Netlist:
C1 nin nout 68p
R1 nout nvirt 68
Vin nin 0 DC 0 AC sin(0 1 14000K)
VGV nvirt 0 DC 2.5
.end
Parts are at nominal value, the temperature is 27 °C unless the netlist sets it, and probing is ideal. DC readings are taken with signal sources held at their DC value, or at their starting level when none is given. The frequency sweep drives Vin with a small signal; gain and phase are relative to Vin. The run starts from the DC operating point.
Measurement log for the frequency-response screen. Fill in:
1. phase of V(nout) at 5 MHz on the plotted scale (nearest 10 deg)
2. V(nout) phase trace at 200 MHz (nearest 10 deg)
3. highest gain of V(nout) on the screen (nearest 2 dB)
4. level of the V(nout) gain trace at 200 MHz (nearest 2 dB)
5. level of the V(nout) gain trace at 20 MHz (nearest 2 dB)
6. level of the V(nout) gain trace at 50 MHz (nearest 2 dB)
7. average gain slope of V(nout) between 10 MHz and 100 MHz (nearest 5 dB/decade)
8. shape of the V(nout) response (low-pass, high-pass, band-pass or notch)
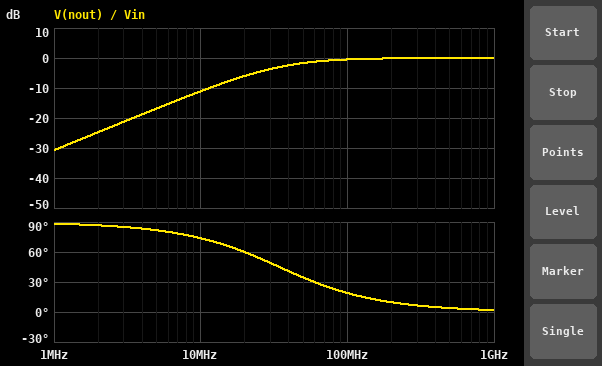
80 deg
10 deg
0 dB
0 dB
-6 dB
-2 dB
10 dB/decade
high-pass
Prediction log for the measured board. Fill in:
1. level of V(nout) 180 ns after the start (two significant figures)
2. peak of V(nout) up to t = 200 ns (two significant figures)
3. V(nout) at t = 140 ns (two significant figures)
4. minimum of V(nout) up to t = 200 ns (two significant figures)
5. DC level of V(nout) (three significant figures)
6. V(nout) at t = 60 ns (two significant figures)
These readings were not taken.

2.1 V
2.9 V
2.8 V
2.1 V
2.50 V
2.6 V
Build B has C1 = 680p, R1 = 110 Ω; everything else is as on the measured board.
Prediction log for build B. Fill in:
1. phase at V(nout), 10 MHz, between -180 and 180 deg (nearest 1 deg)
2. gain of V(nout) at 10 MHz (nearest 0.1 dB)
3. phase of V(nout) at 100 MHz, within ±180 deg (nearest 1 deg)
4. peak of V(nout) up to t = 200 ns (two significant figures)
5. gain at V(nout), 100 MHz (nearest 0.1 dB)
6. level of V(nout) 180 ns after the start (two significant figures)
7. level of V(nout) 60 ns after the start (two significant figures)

12 deg
-0.2 dB
1 deg
3.5 V
0 dB
2.2 V
1.7 V
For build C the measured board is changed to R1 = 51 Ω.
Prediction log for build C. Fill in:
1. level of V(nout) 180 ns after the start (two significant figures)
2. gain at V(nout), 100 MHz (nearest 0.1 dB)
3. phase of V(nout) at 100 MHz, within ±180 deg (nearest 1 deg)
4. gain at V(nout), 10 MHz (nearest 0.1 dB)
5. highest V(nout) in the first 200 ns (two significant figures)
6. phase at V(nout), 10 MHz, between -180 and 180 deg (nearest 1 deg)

2.2 V
-0.8 dB
25 deg
-13.4 dB
2.8 V
78 deg
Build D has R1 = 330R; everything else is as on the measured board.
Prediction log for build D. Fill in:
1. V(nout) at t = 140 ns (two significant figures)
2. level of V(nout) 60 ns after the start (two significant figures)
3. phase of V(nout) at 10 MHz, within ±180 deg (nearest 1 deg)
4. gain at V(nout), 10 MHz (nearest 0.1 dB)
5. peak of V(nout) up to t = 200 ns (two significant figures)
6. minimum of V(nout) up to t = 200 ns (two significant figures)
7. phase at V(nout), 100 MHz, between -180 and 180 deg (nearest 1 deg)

2.7 V
2.0 V
35 deg
-1.8 dB
3.4 V
1.6 V
4 deg
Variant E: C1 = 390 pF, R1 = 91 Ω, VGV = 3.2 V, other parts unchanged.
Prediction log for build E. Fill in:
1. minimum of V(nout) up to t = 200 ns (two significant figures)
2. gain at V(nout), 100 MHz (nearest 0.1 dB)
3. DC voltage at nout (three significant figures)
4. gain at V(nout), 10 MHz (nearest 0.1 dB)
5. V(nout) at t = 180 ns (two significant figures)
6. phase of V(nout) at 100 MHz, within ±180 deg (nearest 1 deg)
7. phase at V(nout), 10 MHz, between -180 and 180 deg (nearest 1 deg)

2.2 V
0 dB
3.20 V
-0.8 dB
2.8 V
3 deg
24 deg
